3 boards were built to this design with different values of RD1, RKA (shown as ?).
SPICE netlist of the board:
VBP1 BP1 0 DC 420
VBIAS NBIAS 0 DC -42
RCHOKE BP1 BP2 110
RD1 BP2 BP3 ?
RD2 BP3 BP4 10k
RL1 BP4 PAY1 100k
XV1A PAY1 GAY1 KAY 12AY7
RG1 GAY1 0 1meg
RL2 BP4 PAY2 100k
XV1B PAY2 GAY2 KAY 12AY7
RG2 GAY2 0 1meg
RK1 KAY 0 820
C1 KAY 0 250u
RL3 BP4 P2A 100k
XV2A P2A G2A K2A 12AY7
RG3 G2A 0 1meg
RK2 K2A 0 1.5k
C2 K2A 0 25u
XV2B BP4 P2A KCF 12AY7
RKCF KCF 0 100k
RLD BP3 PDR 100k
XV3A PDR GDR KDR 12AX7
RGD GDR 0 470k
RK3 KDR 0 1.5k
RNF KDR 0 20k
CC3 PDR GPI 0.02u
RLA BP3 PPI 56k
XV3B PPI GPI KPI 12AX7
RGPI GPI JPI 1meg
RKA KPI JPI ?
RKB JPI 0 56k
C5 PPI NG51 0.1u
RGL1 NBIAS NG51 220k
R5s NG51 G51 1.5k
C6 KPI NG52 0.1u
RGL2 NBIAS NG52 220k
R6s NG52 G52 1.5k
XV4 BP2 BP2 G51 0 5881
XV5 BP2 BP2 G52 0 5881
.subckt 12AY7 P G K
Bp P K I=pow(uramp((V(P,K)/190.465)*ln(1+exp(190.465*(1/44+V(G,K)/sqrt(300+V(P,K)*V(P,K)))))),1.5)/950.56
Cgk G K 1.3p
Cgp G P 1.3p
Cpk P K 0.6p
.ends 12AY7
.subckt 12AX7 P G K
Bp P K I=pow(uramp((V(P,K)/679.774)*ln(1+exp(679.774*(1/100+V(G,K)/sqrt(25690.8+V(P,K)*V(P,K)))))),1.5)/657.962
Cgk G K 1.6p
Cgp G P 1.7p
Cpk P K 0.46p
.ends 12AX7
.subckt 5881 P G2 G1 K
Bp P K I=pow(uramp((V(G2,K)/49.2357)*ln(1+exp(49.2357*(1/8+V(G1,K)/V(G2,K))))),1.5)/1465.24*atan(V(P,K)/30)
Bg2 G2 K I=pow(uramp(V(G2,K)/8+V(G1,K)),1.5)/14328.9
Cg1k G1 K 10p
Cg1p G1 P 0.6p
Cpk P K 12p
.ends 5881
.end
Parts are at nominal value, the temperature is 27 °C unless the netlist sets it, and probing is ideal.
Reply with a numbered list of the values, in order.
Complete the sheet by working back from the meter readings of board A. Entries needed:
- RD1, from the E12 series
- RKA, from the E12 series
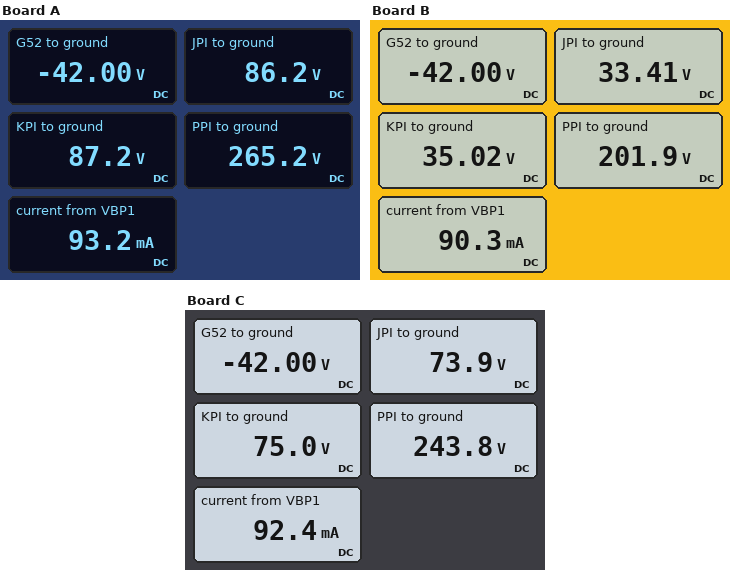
1. 6.8 kΩ
2. 680 Ω
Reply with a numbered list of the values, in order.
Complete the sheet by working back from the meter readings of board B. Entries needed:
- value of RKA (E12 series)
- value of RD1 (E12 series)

1. 2.7 kΩ
2. 33 kΩ
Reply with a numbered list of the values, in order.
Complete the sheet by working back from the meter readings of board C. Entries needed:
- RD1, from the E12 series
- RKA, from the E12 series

1. 12 kΩ
2. 820 Ω
